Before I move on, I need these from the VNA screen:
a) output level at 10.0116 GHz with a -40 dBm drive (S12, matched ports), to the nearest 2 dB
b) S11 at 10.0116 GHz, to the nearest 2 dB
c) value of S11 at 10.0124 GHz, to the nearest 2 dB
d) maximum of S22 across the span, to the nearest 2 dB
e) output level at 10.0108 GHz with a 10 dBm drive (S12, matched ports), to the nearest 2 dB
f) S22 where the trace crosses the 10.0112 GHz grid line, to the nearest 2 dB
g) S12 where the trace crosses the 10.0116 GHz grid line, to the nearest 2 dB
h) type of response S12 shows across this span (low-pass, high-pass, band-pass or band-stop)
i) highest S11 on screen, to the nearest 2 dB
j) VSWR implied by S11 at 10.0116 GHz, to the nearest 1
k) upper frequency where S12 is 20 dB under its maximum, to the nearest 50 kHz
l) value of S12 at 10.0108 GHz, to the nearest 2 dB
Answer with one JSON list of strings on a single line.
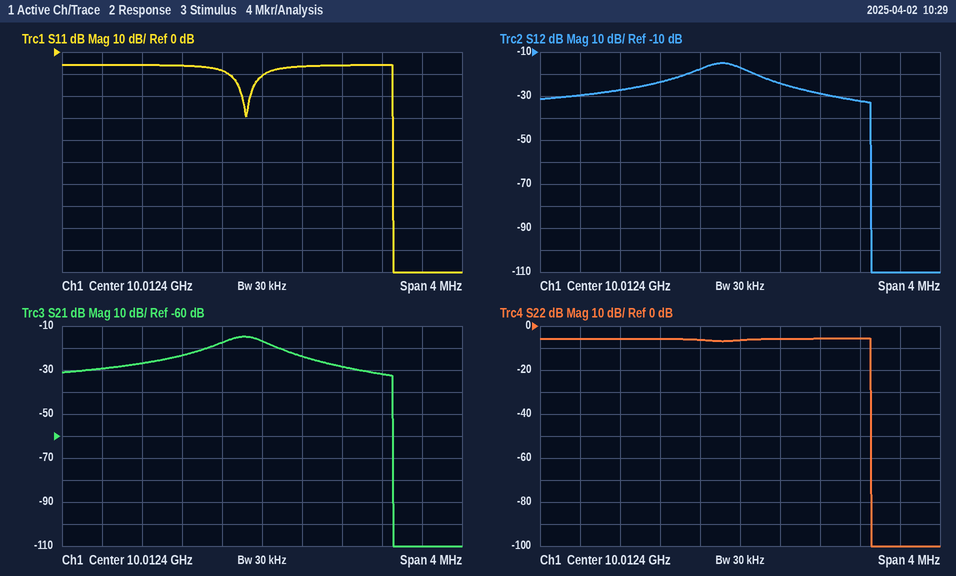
["-64 dBm", "-6 dB", "-10 dB", "-6 dB", "-20 dBm", "-6 dB", "-24 dB", "band-pass", "-6 dB", "3", "10.01370 GHz", "-30 dB"]
